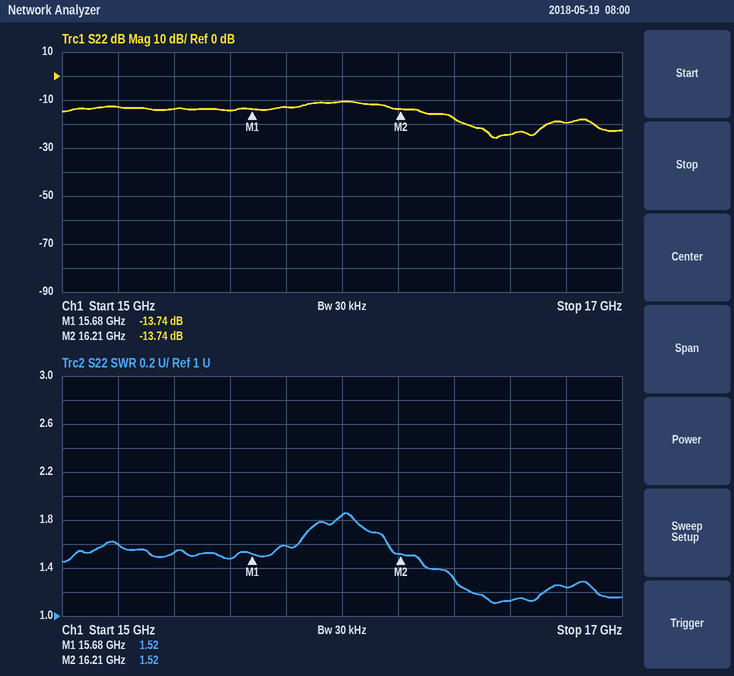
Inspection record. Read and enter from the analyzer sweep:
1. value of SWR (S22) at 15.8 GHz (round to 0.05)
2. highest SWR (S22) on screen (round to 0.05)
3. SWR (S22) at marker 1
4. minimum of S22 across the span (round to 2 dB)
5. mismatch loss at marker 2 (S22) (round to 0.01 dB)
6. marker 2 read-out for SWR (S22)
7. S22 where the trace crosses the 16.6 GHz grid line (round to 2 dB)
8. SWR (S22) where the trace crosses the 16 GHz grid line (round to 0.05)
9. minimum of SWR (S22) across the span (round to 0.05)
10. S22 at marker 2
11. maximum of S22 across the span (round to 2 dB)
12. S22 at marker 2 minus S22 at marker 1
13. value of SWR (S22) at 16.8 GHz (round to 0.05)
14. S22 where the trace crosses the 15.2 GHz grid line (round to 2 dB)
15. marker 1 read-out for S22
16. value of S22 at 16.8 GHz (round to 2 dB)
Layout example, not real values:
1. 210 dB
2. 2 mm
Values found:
1. 1.60
2. 1.85
3. 1.52
4. -26 dB
5. 0.19 dB
6. 1.52
7. -24 dB
8. 1.85
9. 1.10
10. -13.74 dB
11. -10 dB
12. 0.00 dB
13. 1.25
14. -12 dB
15. -13.74 dB
16. -20 dB
